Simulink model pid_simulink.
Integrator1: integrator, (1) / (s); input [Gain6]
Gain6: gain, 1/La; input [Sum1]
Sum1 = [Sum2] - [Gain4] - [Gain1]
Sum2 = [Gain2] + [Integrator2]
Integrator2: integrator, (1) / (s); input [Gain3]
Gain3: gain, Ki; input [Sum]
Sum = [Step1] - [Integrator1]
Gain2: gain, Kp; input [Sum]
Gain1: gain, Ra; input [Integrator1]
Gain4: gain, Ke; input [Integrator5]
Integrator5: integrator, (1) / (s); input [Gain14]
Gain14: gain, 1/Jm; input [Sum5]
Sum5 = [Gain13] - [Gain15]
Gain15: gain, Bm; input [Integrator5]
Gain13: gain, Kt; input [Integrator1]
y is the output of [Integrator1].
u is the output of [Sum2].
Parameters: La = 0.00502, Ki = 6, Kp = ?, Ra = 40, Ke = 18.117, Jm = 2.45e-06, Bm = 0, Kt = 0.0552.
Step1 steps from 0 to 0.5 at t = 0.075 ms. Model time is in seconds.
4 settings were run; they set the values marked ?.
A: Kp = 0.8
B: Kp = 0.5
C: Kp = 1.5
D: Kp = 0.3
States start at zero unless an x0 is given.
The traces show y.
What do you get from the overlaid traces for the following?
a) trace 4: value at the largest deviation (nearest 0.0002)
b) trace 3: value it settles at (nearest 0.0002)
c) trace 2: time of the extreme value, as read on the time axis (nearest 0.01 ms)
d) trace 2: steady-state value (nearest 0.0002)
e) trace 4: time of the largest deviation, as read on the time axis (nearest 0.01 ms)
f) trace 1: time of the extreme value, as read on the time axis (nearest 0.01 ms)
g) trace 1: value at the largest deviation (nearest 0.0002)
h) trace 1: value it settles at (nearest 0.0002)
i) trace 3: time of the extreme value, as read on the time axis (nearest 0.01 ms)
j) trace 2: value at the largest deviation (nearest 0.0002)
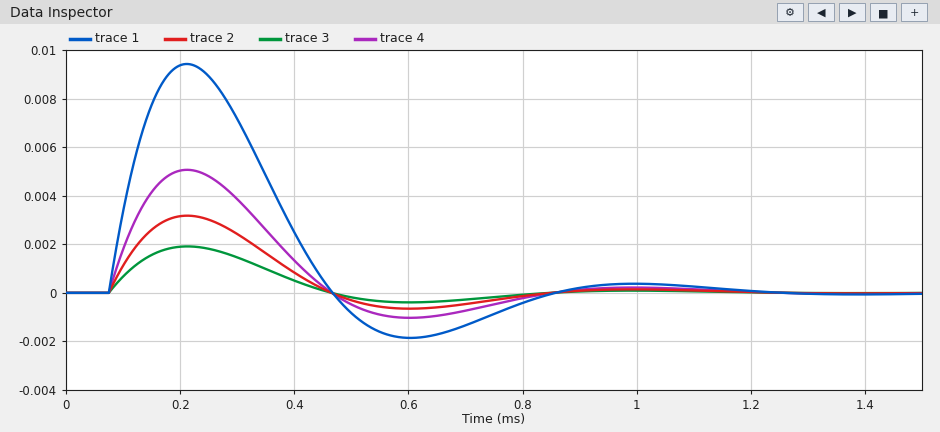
0.0050
0.0000
0.21 ms
0.0000
0.21 ms
0.21 ms
0.0094
0.0000
0.21 ms
0.0032
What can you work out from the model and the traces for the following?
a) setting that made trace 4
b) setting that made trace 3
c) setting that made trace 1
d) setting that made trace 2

A
D
C
B
